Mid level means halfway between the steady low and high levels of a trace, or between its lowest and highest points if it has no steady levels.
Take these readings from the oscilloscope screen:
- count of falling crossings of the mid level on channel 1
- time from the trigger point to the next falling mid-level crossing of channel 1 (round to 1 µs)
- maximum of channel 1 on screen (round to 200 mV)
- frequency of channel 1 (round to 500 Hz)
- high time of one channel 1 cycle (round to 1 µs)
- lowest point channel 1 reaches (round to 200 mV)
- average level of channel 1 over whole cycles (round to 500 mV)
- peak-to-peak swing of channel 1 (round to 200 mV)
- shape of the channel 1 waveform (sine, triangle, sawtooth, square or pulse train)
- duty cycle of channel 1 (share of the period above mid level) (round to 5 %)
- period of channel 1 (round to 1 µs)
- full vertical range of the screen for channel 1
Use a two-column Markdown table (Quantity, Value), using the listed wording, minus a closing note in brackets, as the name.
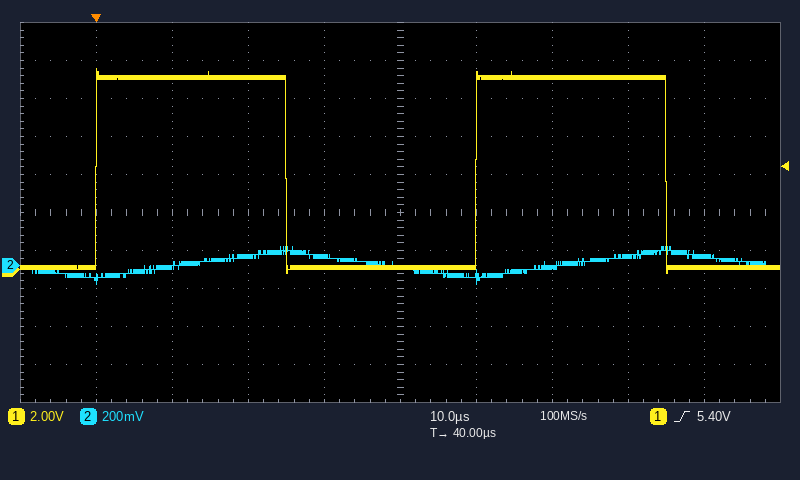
| Quantity | Value |
|---|---|
| count of falling crossings of the mid level on channel 1 | 2 |
| time from the trigger point to the next falling mid-level crossing of channel 1 | 25 µs |
| maximum of channel 1 on screen | 10.6 V |
| frequency of channel 1 | 20.0 kHz |
| high time of one channel 1 cycle | 25 µs |
| lowest point channel 1 reaches | -200 mV |
| average level of channel 1 over whole cycles | 5.0 V |
| peak-to-peak swing of channel 1 | 10.8 V |
| shape of the channel 1 waveform | square |
| duty cycle of channel 1 (share of the period above mid level) | 50 % |
| period of channel 1 | 50 µs |
| full vertical range of the screen for channel 1 | 20 V |
